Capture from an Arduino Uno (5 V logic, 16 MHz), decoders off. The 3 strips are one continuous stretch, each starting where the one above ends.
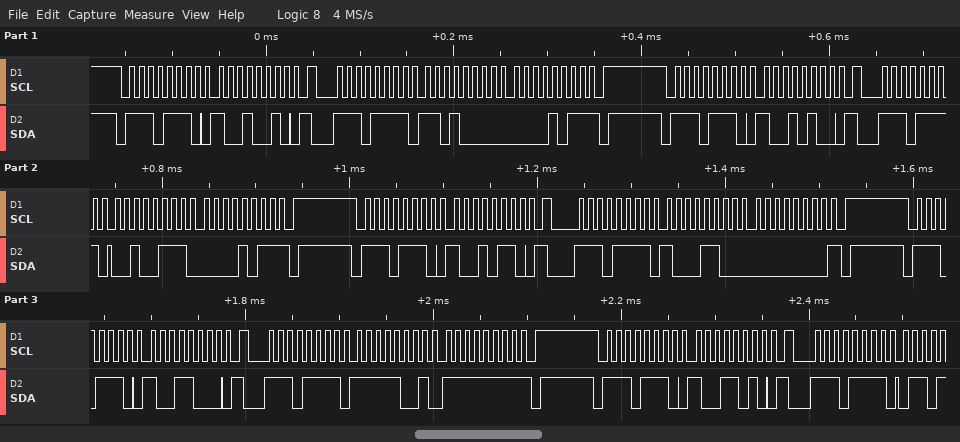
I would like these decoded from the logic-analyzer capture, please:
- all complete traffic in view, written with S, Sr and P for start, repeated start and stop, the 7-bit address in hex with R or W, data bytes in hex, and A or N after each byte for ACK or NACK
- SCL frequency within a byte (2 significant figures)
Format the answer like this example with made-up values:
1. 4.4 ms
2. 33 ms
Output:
1. S 77W A 92 A Sr 77R A D0 A 0B N P S 77W A 94 A Sr 77R A 27 A 0B N P S 77W A 96 A Sr 77R A 8C A 00 N P S 77W A 98 A Sr 77R A F9 A FF N P S 77W A 9A A Sr 77R A
2. 100 kHz
